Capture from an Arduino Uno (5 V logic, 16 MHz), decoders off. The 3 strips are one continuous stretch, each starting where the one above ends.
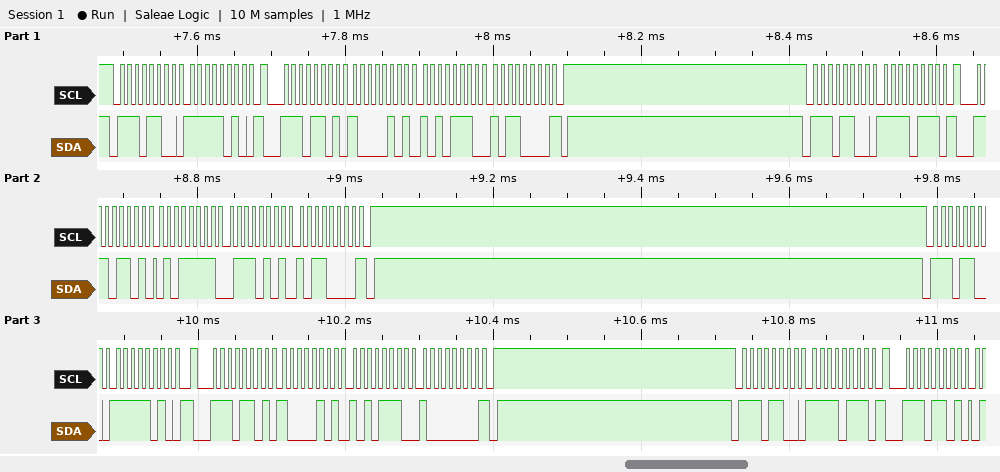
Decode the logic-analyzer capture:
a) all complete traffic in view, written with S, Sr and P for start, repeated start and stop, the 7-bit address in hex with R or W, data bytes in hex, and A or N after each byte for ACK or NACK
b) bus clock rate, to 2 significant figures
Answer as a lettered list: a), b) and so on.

a) S 76W A FA A Sr 76R A 85 A AE A B0 N P S 76W A F7 A Sr 76R A 5F A 75 A B0 N P S 76W A FA A Sr 76R A 85 A AE A 80 N P S 76W A F7 A Sr 76R A
b) 100 kHz
